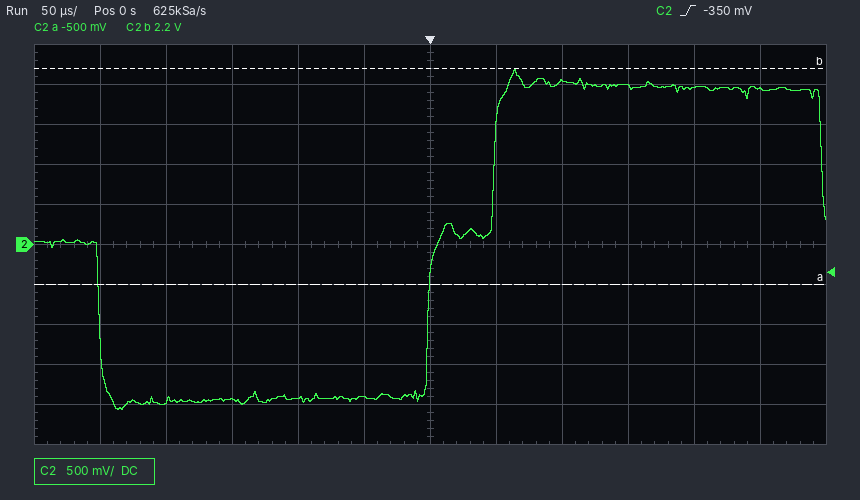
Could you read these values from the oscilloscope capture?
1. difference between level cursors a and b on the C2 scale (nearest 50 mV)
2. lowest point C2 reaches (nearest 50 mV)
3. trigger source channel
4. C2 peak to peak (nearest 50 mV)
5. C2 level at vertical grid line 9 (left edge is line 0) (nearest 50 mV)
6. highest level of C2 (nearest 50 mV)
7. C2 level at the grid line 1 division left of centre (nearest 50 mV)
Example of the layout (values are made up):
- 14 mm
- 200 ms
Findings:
- 2.70 V
- -2.05 V
- C2
- 4.25 V
- 1.95 V
- 2.20 V
- -1.90 V
